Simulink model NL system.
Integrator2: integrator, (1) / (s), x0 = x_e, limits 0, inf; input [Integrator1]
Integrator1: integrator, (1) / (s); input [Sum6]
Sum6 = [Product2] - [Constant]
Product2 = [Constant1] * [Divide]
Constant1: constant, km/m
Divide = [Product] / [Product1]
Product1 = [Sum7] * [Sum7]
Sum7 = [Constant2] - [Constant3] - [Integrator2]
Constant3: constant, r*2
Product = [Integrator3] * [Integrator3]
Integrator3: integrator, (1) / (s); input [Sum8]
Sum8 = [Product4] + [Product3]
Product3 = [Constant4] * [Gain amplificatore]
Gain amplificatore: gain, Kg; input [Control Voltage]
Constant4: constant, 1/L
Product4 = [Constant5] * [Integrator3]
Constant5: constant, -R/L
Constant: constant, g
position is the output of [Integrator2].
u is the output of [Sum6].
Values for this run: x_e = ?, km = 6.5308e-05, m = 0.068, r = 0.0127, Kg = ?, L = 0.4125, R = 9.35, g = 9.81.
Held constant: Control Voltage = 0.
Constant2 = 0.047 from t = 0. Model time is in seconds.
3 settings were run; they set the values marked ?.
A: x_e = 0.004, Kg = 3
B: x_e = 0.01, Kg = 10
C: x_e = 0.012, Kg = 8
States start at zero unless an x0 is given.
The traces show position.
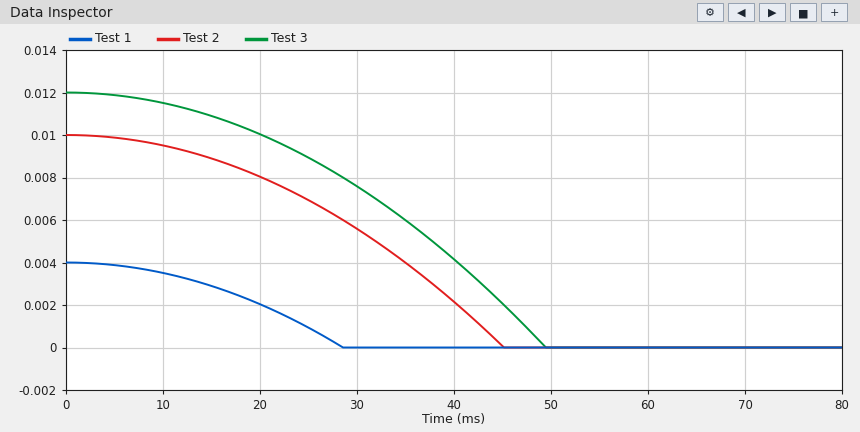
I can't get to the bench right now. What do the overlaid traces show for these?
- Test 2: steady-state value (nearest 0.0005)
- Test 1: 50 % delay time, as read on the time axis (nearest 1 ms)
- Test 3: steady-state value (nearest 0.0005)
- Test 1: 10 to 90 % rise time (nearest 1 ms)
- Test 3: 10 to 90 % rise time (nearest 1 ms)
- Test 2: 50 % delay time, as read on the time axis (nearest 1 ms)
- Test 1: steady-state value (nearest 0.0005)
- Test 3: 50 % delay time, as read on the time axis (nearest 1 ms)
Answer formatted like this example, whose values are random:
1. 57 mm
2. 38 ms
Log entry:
1. 0.0000
2. 20 ms
3. 0.0000
4. 18 ms
5. 31 ms
6. 32 ms
7. 0.0000
8. 35 ms
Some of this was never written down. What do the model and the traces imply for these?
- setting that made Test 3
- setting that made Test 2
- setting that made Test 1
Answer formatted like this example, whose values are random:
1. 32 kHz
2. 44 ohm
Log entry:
1. C
2. B
3. A
